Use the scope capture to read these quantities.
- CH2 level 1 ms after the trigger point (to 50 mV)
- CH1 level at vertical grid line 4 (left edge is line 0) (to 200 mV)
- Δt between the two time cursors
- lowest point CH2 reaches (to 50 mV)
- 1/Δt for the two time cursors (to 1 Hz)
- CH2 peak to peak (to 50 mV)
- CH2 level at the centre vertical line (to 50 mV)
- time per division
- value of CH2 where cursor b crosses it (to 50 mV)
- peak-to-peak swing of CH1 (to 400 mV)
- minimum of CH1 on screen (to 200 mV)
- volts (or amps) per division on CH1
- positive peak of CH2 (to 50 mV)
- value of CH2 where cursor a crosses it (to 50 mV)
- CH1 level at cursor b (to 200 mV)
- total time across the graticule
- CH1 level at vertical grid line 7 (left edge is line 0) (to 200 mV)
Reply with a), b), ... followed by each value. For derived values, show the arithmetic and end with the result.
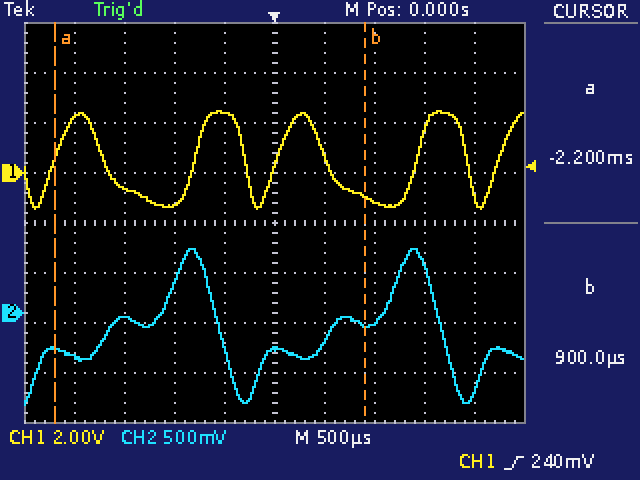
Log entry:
a) -100 mV
b) 2.4 V
c) 900 µs − (-2.2 ms) = 3.10 ms
d) -900 mV
e) 1 / 3.10 ms ≈ 323 Hz
f) 650 mV − (-900 mV) = 1.55 V
g) -350 mV
h) 500 µs
i) -100 mV
j) 4.0 V
k) -1.4 V
l) 2 V
m) 650 mV
n) -350 mV
o) -1.0 V
p) 5 ms
q) -1.2 V
